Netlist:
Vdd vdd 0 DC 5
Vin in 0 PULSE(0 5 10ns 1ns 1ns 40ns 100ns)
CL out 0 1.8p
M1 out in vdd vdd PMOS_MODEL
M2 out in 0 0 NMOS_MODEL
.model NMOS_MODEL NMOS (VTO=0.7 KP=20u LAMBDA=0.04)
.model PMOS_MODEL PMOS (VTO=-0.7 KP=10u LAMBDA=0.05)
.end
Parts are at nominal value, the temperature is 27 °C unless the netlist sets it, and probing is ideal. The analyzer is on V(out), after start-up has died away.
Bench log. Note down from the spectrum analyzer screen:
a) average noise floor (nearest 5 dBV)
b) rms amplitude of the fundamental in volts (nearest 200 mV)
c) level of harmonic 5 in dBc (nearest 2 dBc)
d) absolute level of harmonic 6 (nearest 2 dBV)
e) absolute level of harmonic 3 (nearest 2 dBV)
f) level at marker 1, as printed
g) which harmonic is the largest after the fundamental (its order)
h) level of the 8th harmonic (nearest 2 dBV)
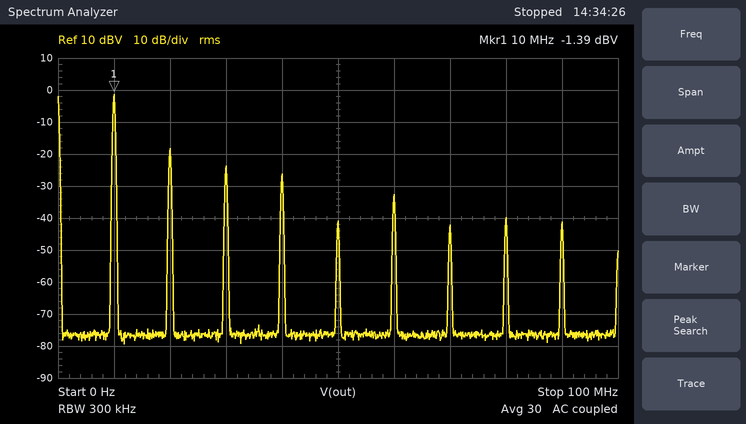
-75 dBV
800 mV
-40 dBc
-32 dBV
-24 dBV
-1.39 dBV
2
-40 dBV
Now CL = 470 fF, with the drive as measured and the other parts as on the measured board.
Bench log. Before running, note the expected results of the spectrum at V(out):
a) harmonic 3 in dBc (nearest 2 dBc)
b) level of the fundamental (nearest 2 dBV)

-16 dBc
6 dBV
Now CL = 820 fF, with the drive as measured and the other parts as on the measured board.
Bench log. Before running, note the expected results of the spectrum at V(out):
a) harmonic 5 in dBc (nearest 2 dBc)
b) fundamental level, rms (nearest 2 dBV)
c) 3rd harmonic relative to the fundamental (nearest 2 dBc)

-36 dBc
4 dBV
-20 dBc
